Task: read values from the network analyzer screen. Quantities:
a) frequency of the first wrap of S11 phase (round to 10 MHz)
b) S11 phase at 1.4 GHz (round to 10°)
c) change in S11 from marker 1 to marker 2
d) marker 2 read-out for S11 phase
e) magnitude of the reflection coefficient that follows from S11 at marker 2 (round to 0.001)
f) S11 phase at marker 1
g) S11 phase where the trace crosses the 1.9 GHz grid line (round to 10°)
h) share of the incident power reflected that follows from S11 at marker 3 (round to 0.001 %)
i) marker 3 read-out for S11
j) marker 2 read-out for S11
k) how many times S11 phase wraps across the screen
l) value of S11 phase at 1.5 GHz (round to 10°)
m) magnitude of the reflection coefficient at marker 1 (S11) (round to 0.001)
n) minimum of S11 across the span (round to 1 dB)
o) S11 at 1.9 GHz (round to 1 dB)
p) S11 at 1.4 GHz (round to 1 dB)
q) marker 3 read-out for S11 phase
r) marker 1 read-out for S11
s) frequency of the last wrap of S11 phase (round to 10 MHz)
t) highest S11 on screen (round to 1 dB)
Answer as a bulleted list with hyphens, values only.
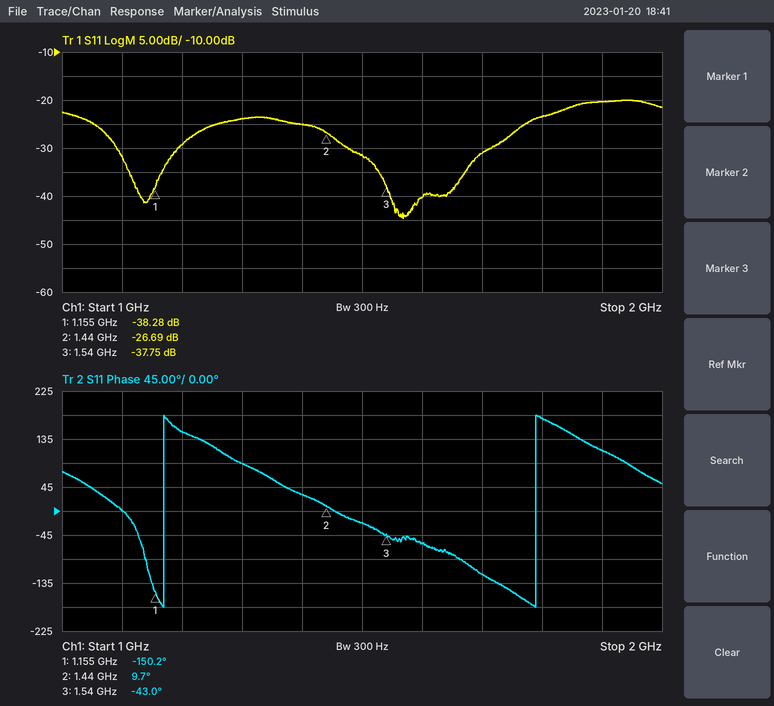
- 1.17 GHz
- 30°
- 11.59 dB
- 9.7°
- 0.046
- -150.2°
- 110°
- 0.017 %
- -37.75 dB
- -26.69 dB
- 2
- -20°
- 0.012
- -45 dB
- -20 dB
- -25 dB
- -43.0°
- -38.28 dB
- 1.79 GHz
- -20 dB
